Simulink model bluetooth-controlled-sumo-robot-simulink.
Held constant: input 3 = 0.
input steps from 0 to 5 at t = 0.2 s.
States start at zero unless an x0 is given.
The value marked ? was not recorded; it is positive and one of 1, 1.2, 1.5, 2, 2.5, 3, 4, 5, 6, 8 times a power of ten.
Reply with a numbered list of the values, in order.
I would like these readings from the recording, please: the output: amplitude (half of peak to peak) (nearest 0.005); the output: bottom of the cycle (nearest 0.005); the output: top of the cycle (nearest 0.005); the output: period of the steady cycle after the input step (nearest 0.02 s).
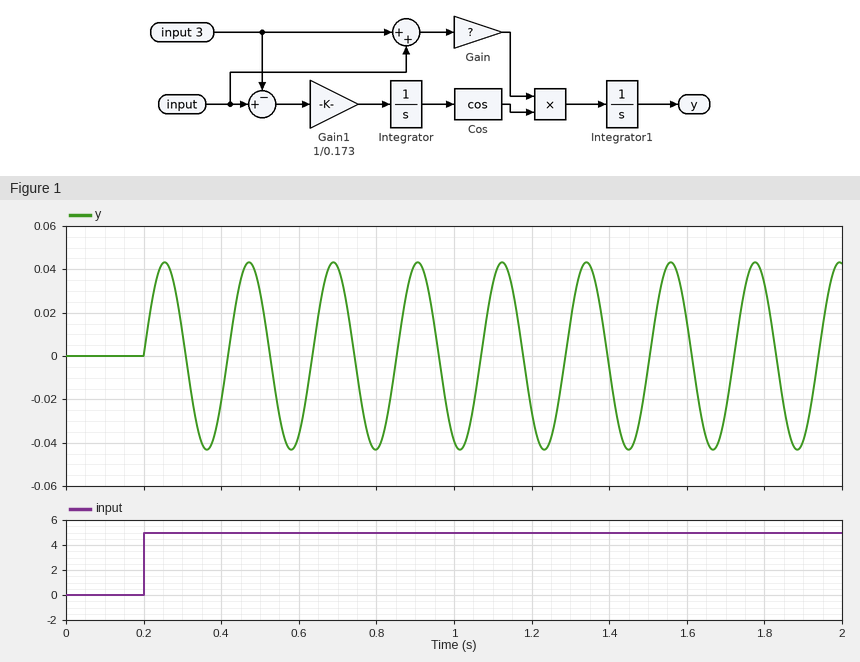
1. 0.045
2. -0.045
3. 0.045
4. 0.22 s
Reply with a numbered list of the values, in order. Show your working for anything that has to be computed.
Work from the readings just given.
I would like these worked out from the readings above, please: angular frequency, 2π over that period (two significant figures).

1. 2π / 0.22 = 29 rad/s
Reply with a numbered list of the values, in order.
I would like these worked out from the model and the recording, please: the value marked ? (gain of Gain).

1. 0.25
